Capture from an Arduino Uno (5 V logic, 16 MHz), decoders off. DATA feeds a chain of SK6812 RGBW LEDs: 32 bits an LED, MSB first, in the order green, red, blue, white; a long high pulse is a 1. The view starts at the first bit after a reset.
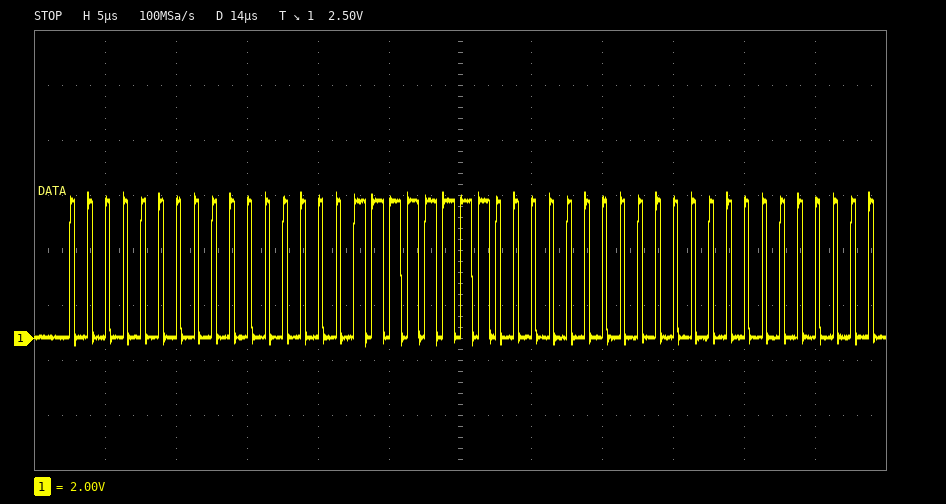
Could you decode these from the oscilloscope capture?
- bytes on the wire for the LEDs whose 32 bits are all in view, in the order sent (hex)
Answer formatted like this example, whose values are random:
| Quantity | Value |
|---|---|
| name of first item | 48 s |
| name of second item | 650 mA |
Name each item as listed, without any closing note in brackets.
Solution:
| Quantity | Value |
|---|---|
| bytes on the wire for the LEDs whose 32 bits are all in view, in the order sent | 00 00 FF 00 |
